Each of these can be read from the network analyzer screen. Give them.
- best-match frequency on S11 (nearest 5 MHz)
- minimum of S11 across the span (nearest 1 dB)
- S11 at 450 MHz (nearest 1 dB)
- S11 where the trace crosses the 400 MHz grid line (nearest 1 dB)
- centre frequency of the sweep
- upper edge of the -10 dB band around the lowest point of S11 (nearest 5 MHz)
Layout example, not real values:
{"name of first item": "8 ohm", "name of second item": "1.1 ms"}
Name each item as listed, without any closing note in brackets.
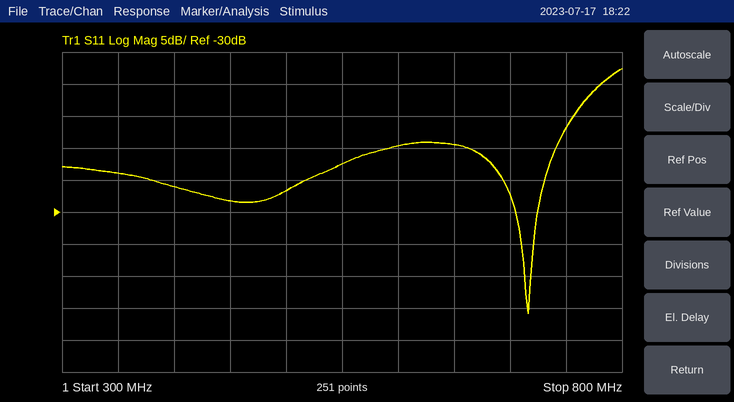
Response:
{"best-match frequency on S11": "715 MHz", "minimum of S11 across the span": "-46 dB", "S11 at 450 MHz": "-28 dB", "S11 where the trace crosses the 400 MHz grid line": "-26 dB", "centre frequency of the sweep": "550 MHz", "upper edge of the -10 dB band around the lowest point of S11": "780 MHz"}
